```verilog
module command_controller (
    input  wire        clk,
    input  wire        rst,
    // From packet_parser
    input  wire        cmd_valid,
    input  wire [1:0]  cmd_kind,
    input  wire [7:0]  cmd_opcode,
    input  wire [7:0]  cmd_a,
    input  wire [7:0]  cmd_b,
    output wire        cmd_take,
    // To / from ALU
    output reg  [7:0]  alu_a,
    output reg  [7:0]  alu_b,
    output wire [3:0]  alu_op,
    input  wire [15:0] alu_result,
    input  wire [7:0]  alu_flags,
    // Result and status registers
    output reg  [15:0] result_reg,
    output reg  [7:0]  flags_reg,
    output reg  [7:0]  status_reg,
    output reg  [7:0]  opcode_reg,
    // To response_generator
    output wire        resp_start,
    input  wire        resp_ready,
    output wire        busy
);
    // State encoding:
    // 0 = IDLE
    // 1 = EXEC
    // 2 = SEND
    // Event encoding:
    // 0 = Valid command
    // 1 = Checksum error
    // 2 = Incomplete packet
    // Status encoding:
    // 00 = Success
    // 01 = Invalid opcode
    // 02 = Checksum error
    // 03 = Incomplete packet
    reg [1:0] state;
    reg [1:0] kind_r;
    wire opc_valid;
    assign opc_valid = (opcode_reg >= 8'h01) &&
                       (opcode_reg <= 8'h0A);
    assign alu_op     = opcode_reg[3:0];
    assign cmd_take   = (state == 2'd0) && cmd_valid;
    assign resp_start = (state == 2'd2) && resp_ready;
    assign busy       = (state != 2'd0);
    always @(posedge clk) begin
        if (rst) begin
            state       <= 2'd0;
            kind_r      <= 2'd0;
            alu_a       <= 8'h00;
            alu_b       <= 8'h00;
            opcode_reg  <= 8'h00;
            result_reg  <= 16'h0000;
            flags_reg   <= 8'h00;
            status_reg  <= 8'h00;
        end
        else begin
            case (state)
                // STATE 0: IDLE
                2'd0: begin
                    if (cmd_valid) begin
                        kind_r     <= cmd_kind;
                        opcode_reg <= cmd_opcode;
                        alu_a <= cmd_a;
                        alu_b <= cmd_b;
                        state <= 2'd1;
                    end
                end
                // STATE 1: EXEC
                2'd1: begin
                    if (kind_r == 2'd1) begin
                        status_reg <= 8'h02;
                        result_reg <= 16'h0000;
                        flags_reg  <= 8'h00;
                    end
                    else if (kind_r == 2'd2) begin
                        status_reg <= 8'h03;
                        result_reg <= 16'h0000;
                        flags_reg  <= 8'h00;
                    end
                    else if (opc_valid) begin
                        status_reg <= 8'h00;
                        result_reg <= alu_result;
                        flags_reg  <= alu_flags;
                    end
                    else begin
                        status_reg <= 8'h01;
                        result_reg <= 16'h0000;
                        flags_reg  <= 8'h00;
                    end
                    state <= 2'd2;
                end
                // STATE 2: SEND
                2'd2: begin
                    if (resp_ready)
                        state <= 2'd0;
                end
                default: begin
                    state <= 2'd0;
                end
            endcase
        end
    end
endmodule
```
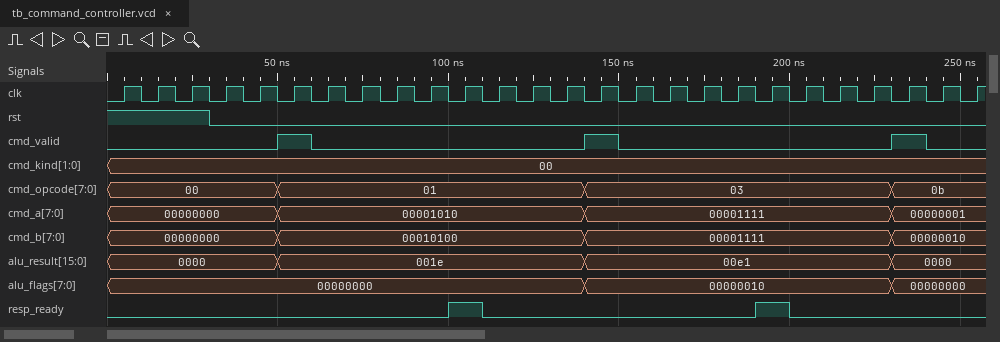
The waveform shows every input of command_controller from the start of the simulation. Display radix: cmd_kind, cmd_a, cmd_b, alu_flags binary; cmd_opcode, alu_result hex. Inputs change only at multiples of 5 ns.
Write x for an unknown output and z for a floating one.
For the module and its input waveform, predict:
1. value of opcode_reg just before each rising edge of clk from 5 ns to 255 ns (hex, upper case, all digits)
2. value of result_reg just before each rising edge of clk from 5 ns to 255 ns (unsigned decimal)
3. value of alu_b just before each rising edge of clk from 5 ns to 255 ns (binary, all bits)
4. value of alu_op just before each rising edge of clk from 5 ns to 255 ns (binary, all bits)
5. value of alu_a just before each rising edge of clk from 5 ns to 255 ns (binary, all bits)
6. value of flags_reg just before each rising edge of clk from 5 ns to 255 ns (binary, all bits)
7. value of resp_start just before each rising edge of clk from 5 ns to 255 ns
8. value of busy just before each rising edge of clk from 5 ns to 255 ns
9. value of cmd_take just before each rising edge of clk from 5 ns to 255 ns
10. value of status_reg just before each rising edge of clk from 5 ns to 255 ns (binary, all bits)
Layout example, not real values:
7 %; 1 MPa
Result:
x, 00, 00, 00, 00, 00, 01, 01, 01, 01, 01, 01, 01, 01, 01, 03, 03, 03, 03, 03, 03, 03, 03, 03, 0B, 0B; x, 0, 0, 0, 0, 0, 0, 30, 30, 30, 30, 30, 30, 30, 30, 30, 225, 225, 225, 225, 225, 225, 225, 225, 225, 0; x, 00000000, 00000000, 00000000, 00000000, 00000000, 00010100, 00010100, 00010100, 00010100, 00010100, 00010100, 00010100, 00010100, 00010100, 00001111, 00001111, 00001111, 00001111, 00001111, 00001111, 00001111, 00001111, 00001111, 00000010, 00000010; x, 0000, 0000, 0000, 0000, 0000, 0001, 0001, 0001, 0001, 0001, 0001, 0001, 0001, 0001, 0011, 0011, 0011, 0011, 0011, 0011, 0011, 0011, 0011, 1011, 1011; x, 00000000, 00000000, 00000000, 00000000, 00000000, 00001010, 00001010, 00001010, 00001010, 00001010, 00001010, 00001010, 00001010, 00001010, 00001111, 00001111, 00001111, 00001111, 00001111, 00001111, 00001111, 00001111, 00001111, 00000001, 00000001; x, 00000000, 00000000, 00000000, 00000000, 00000000, 00000000, 00000000, 00000000, 00000000, 00000000, 00000000, 00000000, 00000000, 00000000, 00000000, 00000010, 00000010, 00000010, 00000010, 00000010, 00000010, 00000010, 00000010, 00000010, 00000000; 0 0 0 0 0 0 0 0 0 0 1 0 0 0 0 0 0 0 0 1 0 0 0 0 0 0; x 0 0 0 0 0 1 1 1 1 1 0 0 0 0 1 1 1 1 1 0 0 0 0 1 1; 0 0 0 0 0 1 0 0 0 0 0 0 0 0 1 0 0 0 0 0 0 0 0 1 0 0; x, 00000000, 00000000, 00000000, 00000000, 00000000, 00000000, 00000000, 00000000, 00000000, 00000000, 00000000, 00000000, 00000000, 00000000, 00000000, 00000000, 00000000, 00000000, 00000000, 00000000, 00000000, 00000000, 00000000, 00000000, 00000001
